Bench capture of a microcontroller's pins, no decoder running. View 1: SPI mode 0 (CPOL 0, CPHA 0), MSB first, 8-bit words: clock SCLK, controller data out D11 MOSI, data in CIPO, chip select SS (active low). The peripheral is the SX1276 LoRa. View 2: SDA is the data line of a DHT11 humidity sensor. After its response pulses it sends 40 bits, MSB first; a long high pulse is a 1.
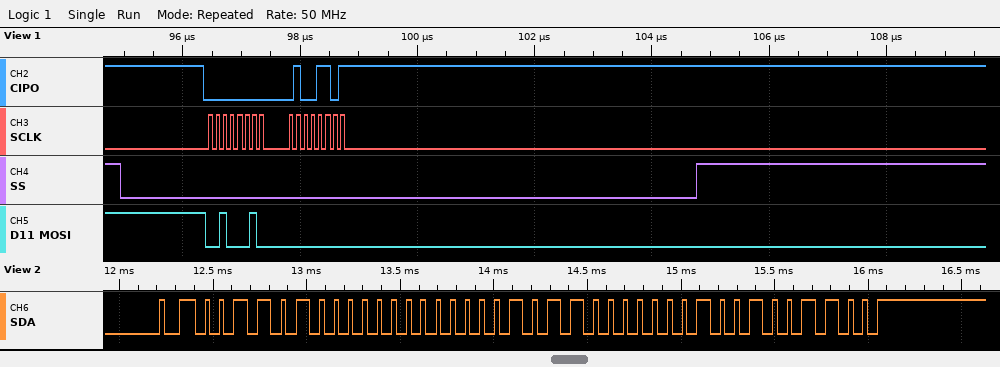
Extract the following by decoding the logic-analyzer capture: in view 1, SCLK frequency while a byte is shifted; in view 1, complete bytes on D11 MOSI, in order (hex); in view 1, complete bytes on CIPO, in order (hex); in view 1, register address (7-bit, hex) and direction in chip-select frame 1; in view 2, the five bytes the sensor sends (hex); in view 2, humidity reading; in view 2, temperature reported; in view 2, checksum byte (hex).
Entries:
8 MHz
22 00
00 4D
0x22 read
34 00 16 02 4C
52 %
22.2 °C
0x4C
